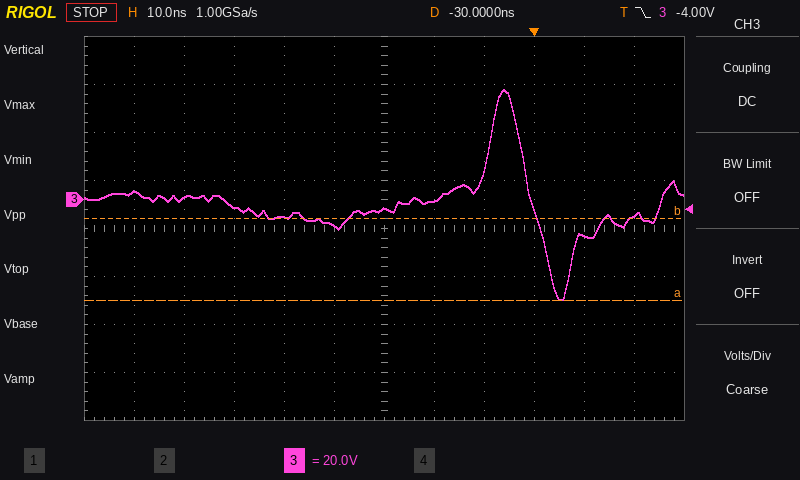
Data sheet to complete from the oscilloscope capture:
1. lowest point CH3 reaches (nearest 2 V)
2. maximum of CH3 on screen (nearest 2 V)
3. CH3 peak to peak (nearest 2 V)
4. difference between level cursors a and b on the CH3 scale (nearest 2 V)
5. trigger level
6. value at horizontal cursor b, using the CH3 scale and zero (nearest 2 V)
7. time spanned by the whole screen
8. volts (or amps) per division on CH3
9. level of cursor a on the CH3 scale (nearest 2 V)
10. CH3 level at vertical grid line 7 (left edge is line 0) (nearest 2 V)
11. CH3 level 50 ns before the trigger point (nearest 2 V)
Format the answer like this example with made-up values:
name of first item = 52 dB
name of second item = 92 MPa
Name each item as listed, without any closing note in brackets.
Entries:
lowest point CH3 reaches = -42 V
maximum of CH3 on screen = 46 V
CH3 peak to peak = 88 V
difference between level cursors a and b on the CH3 scale = 34 V
trigger level = -4.00 V
value at horizontal cursor b, using the CH3 scale and zero = -8 V
time spanned by the whole screen = 120 ns
volts (or amps) per division on CH3 = 20 V
level of cursor a on the CH3 scale = -42 V
CH3 level at vertical grid line 7 (left edge is line 0) = 0 V
CH3 level 50 ns before the trigger point = -8 V
